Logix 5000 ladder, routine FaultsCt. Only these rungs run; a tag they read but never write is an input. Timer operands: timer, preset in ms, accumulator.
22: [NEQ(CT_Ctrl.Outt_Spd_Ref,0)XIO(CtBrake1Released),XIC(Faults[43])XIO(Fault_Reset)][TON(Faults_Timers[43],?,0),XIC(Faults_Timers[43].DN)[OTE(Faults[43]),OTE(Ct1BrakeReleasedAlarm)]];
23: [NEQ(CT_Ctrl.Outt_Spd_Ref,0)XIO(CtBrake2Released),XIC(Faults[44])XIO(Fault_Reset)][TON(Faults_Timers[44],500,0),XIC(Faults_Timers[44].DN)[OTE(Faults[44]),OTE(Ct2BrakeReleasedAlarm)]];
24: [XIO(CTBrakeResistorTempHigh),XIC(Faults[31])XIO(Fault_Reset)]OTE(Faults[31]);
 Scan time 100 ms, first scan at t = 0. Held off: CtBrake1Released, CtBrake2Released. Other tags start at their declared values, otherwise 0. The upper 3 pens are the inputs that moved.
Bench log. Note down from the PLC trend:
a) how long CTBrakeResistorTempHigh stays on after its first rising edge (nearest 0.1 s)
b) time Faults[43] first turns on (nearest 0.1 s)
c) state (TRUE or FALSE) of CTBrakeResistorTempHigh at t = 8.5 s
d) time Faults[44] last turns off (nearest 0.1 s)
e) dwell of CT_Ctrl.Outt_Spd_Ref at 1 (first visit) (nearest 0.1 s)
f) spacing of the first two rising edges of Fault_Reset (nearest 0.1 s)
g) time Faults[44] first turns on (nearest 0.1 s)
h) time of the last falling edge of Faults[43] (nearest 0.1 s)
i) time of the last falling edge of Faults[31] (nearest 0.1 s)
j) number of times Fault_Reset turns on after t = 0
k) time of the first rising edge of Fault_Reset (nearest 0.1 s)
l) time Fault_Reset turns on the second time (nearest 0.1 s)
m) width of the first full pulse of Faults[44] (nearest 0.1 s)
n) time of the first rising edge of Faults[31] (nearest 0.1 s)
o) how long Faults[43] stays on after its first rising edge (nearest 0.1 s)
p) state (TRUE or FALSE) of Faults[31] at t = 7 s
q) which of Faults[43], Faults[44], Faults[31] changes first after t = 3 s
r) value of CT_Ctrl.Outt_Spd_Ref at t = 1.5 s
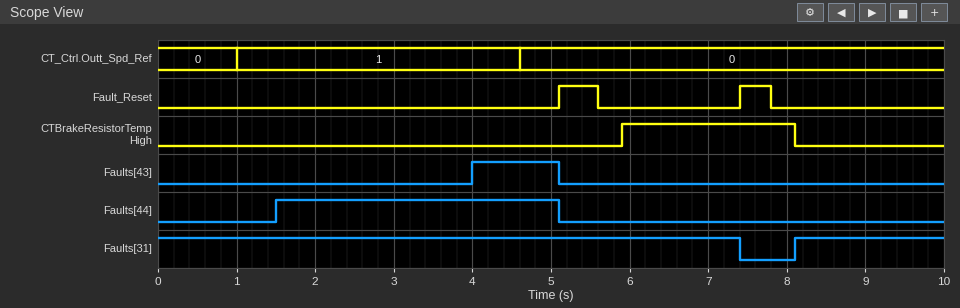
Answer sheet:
2.2 s
4.0 s
FALSE
5.1 s
3.6 s
2.3 s
1.5 s
5.1 s
7.4 s
2
5.1 s
7.4 s
3.6 s
8.1 s
1.1 s
TRUE
Faults[43]
1
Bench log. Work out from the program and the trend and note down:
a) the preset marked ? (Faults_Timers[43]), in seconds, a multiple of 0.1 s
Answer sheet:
3.0 s
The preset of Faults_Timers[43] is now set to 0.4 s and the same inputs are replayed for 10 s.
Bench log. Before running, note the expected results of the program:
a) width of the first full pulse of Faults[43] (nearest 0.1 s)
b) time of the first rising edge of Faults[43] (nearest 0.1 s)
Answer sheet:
3.7 s
1.4 s
